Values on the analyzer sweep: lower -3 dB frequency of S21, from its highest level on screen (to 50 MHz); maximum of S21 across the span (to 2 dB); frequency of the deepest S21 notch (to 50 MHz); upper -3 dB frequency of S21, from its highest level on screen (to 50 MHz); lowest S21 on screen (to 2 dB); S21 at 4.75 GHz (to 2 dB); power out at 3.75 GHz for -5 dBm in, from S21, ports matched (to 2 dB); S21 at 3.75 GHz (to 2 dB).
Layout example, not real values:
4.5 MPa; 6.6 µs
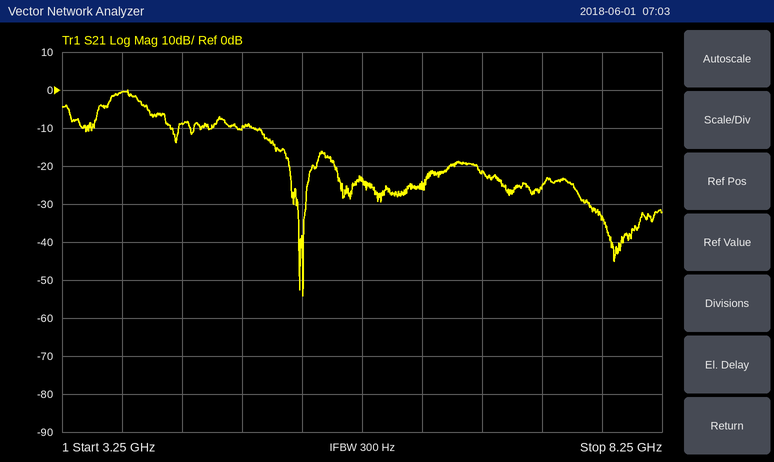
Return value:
3.65 GHz; 0 dB; 5.25 GHz; 3.90 GHz; -54 dB; -10 dB; -6 dBm; 0 dB
